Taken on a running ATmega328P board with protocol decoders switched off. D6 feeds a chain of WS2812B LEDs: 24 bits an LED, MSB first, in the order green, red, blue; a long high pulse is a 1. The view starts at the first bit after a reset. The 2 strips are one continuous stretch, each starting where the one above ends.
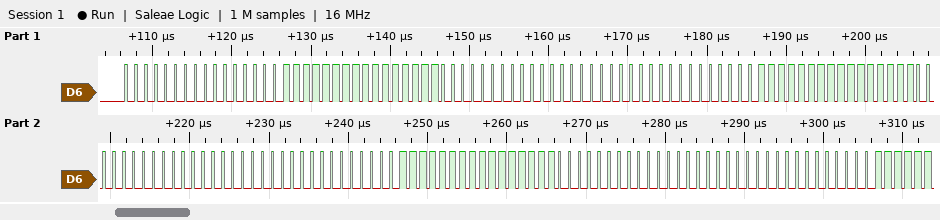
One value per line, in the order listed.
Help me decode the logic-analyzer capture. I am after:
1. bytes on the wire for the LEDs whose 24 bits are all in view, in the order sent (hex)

00 00 FF FF 00 00 00 00 FF FF 00 00 00 00 FF FF 00 00
